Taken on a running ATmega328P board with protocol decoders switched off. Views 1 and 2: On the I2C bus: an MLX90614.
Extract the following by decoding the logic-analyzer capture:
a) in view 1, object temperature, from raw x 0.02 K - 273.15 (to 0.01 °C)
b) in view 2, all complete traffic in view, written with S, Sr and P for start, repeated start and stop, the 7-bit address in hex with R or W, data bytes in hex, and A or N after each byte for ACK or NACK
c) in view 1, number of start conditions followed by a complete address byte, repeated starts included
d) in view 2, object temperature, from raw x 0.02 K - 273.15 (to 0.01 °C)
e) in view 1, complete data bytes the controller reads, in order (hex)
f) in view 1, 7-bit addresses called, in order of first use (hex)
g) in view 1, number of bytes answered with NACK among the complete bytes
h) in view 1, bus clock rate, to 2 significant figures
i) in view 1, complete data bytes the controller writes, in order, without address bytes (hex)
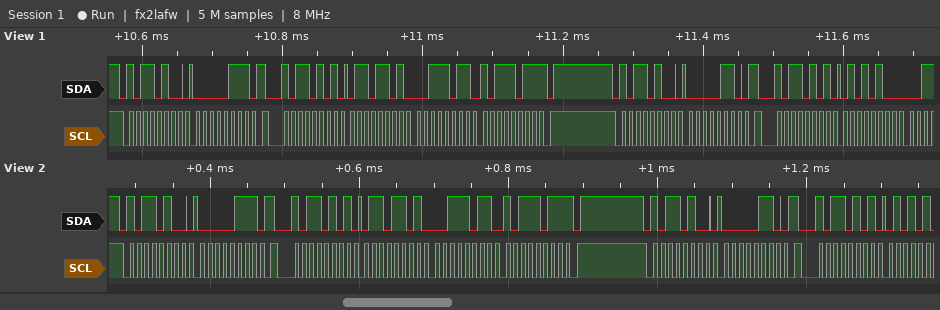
31.11 °C
S 5AW A 07 A Sr 5AR A 6D A 3B A BB N P S 5AW A 06 A Sr 5AR A
4
31.11 °C
6D 3B BB 54
0x5A
1
100 kHz
07 06
